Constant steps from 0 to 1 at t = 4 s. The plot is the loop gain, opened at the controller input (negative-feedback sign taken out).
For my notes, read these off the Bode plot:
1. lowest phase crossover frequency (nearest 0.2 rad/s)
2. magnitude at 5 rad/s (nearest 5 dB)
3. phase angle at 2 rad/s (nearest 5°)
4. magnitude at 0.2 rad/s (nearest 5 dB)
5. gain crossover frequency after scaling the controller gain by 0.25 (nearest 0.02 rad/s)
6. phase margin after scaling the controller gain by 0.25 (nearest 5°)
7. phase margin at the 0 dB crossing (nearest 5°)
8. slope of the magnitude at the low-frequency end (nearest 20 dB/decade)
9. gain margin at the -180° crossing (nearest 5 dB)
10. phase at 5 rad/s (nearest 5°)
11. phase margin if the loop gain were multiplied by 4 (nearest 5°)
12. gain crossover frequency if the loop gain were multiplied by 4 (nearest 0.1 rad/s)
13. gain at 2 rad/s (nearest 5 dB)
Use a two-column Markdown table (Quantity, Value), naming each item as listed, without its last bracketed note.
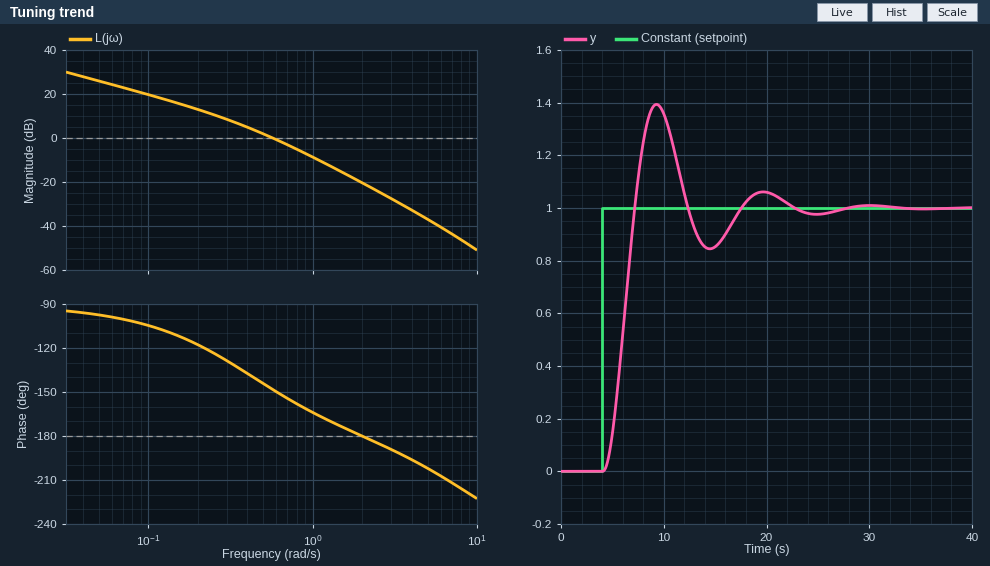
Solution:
| Quantity | Value |
|---|---|
| lowest phase crossover frequency | 2.0 rad/s |
| magnitude at 5 rad/s | -35 dB |
| phase angle at 2 rad/s | -180° |
| magnitude at 0.2 rad/s | 15 dB |
| gain crossover frequency after scaling the controller gain by 0.25 | 0.22 rad/s |
| phase margin after scaling the controller gain by 0.25 | 60° |
| phase margin at the 0 dB crossing | 30° |
| slope of the magnitude at the low-frequency end | -20 dB/decade |
| gain margin at the -180° crossing | 20 dB |
| phase at 5 rad/s | -200° |
| phase margin if the loop gain were multiplied by 4 | 10° |
| gain crossover frequency if the loop gain were multiplied by 4 | 1.2 rad/s |
| gain at 2 rad/s | -20 dB |
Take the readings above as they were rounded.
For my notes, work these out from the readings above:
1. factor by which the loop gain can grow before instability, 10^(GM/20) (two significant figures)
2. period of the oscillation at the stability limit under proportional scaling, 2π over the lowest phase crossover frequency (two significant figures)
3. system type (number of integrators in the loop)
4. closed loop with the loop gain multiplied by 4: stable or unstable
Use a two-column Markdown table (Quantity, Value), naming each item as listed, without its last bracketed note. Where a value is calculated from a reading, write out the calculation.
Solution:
| Quantity | Value |
|---|---|
| factor by which the loop gain can grow before instability, 10^(GM/20) | 10^(20 / 20) = 10 |
| period of the oscillation at the stability limit under proportional scaling, 2π over the lowest phase crossover frequency | 2π / 2 = 3.1 s |
| system type | 1 |
| closed loop with the loop gain multiplied by 4: stable or unstable | stable |
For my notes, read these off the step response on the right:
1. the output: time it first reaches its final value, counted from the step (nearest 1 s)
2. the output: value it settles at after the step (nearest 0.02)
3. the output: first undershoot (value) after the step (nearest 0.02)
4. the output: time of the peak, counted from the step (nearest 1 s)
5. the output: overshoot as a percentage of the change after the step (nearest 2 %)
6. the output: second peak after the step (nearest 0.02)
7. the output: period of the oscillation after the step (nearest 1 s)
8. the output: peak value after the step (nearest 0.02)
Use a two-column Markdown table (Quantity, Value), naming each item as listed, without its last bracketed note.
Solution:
| Quantity | Value |
|---|---|
| the output: time it first reaches its final value, counted from the step | 3 s |
| the output: value it settles at after the step | 1.00 |
| the output: first undershoot (value) after the step | 0.84 |
| the output: time of the peak, counted from the step | 5 s |
| the output: overshoot as a percentage of the change after the step | 40 % |
| the output: second peak after the step | 1.06 |
| the output: period of the oscillation after the step | 10 s |
| the output: peak value after the step | 1.40 |
